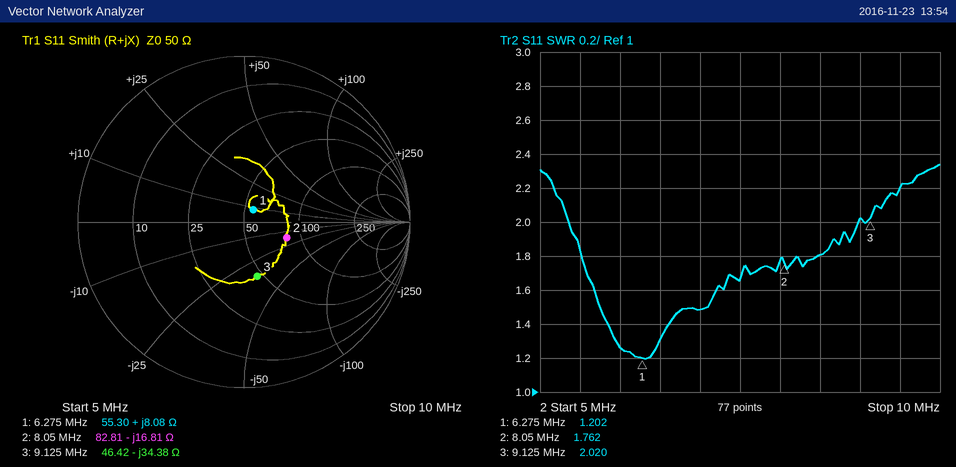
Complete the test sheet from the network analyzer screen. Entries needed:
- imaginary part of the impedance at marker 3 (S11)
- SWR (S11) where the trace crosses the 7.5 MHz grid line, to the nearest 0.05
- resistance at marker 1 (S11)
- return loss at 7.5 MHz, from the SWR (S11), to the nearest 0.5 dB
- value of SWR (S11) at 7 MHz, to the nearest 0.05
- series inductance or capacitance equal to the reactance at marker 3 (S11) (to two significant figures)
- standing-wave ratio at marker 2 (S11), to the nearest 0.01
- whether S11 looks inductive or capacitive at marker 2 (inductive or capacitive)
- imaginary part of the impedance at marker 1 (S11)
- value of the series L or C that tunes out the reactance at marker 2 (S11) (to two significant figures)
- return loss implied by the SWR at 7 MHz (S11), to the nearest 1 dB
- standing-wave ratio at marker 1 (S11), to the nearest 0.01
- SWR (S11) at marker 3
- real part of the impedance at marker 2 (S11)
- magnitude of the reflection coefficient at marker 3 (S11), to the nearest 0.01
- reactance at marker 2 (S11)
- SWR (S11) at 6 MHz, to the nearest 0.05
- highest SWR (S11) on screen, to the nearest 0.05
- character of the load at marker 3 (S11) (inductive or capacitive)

-34.38 Ω
1.65
55.30 Ω
12.0 dB
1.50
510 pF
1.76
capacitive
+8.08 Ω
330 nH
14 dB
1.20
2.020
82.81 Ω
0.34
-16.81 Ω
1.25
2.35
capacitive
